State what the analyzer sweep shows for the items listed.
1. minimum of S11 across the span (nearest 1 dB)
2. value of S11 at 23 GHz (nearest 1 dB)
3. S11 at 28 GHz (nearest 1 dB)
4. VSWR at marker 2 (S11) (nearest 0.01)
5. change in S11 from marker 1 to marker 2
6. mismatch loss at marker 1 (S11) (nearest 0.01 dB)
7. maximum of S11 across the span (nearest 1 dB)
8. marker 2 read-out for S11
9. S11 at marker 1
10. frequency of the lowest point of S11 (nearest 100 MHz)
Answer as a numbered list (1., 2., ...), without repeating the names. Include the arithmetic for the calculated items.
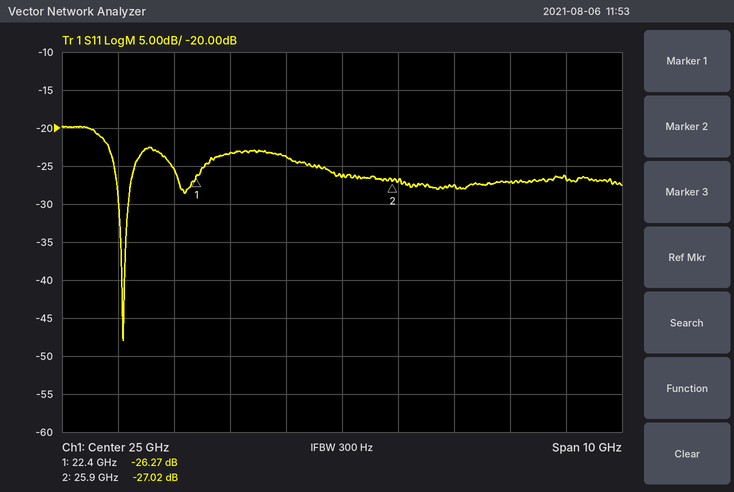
1. -48 dB
2. -23 dB
3. -27 dB
4. (1 + 0.0446)/(1 − 0.0446) ≈ 1.09
5. -27.02 − (-26.27) = -0.75 dB
6. −10 log10(1 − 10^(-26.27/10)) ≈ 0.01 dB
7. -20 dB
8. -27.02 dB
9. -26.27 dB
10. 21.1 GHz
